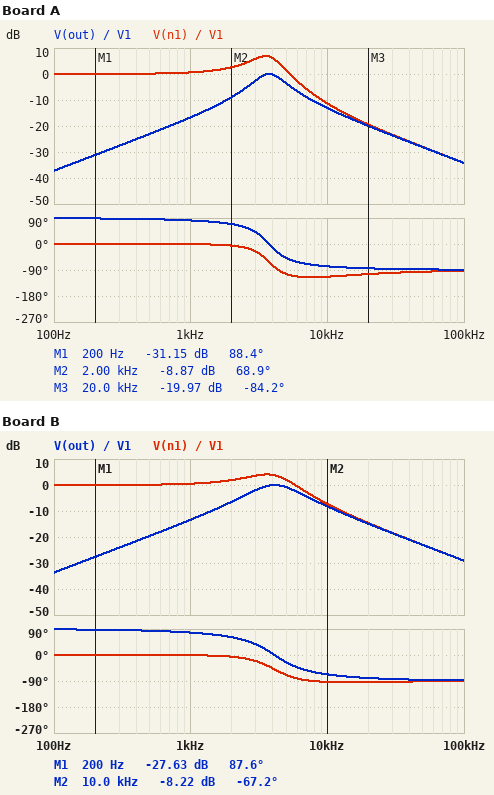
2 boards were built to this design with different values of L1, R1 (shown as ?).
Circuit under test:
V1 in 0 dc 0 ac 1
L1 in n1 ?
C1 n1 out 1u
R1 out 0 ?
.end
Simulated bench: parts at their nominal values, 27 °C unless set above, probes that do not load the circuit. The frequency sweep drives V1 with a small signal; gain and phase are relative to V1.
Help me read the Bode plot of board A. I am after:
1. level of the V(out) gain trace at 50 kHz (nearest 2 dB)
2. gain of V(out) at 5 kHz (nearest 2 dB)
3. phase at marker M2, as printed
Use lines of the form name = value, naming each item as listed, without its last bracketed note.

level of the V(out) gain trace at 50 kHz = -28 dB
gain of V(out) at 5 kHz = -4 dB
phase at marker M2, as printed = 68.9 deg
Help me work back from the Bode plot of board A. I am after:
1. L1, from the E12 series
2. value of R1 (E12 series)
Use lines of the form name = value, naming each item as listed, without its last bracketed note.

L1, from the E12 series = 1.8 mH
value of R1 = 22 Ω
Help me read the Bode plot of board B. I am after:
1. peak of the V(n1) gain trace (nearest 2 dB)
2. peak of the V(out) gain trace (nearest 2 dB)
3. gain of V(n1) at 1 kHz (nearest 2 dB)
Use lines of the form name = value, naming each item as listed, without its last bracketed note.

peak of the V(n1) gain trace = 4 dB
peak of the V(out) gain trace = 0 dB
gain of V(n1) at 1 kHz = 0 dB
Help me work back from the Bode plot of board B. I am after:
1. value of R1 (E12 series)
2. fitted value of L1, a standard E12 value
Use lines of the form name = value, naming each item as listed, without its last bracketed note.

value of R1 = 33 Ω
fitted value of L1, a standard E12 value = 1.5 mH
